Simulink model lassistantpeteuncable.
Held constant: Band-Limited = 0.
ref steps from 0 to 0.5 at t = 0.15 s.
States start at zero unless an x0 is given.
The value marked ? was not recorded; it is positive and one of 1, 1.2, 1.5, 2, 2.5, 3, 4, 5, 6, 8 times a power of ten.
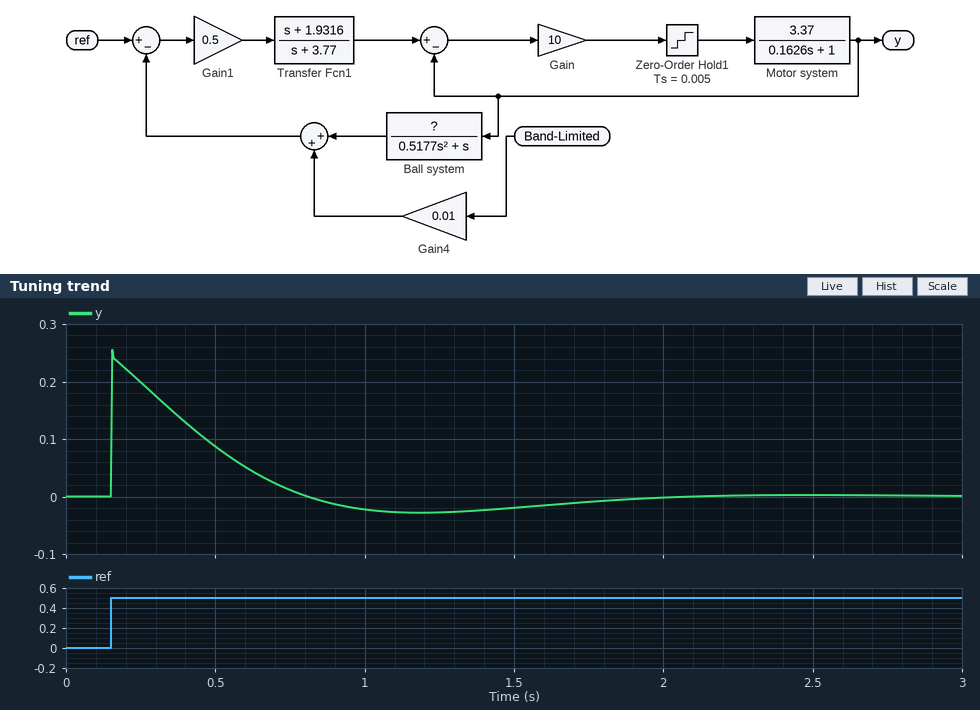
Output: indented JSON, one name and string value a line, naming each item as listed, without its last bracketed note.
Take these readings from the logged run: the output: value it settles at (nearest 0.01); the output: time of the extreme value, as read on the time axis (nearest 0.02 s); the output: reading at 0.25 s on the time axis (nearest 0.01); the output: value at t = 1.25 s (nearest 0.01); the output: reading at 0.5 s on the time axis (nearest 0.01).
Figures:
{
  "the output: value it settles at": "0.00",
  "the output: time of the extreme value, as read on the time axis": "0.16 s",
  "the output: reading at 0.25 s on the time axis": "0.20",
  "the output: value at t = 1.25 s": "-0.03",
  "the output: reading at 0.5 s on the time axis": "0.09"
}
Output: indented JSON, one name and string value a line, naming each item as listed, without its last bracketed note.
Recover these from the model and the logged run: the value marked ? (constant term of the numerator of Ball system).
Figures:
{
  "the value marked ?": "10"
}
